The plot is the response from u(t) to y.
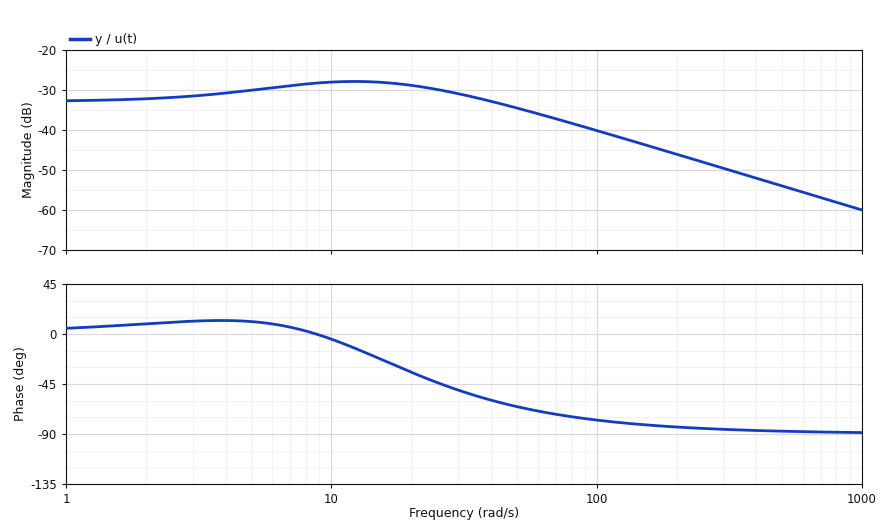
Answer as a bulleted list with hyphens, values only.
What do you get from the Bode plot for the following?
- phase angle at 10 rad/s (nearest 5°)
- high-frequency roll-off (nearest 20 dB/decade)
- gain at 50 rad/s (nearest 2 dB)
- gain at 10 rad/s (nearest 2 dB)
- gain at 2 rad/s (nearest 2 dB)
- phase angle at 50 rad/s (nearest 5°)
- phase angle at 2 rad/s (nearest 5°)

- -5°
- -20 dB/decade
- -34 dB
- -28 dB
- -32 dB
- -65°
- 10°
